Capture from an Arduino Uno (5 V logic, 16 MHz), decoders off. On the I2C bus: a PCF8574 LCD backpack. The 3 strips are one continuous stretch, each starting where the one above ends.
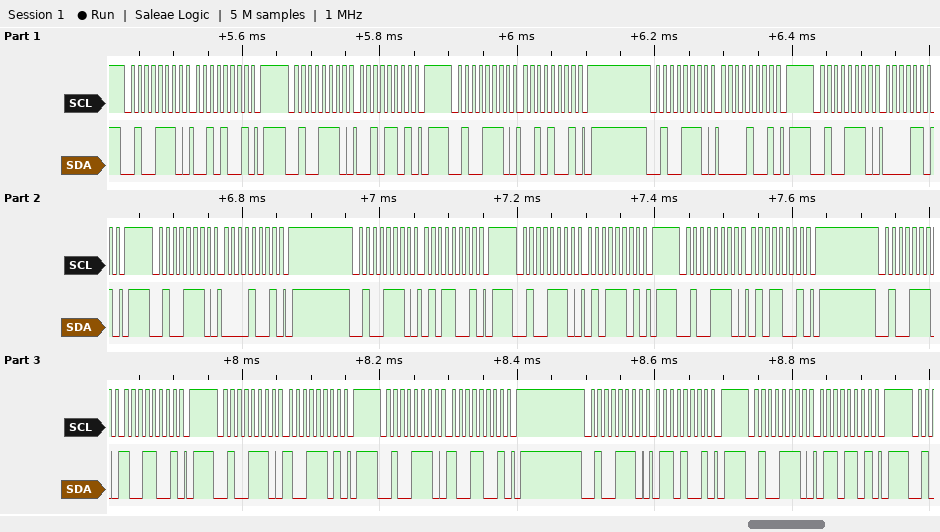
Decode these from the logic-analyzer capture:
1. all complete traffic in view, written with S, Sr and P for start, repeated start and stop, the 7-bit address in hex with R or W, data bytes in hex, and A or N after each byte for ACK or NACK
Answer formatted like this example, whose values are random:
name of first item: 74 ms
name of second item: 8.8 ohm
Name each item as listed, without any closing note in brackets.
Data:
all complete traffic in view, written with S, Sr and P for start, repeated start and stop, the 7-bit address in hex with R or W, data bytes in hex, and A or N after each byte for ACK or NACK: S 27W A 29 A P S 27W A 2D A P S 27W A 29 A P S 27W A 09 A P S 27W A 0D A P S 27W A 09 A P S 27W A 59 A P S 27W A 5D A P S 27W A 59 A P S 27W A 99 A P S 27W A 9D A P S 27W A 99 A P S 27W A 69 A P S 27W A 6D A P
